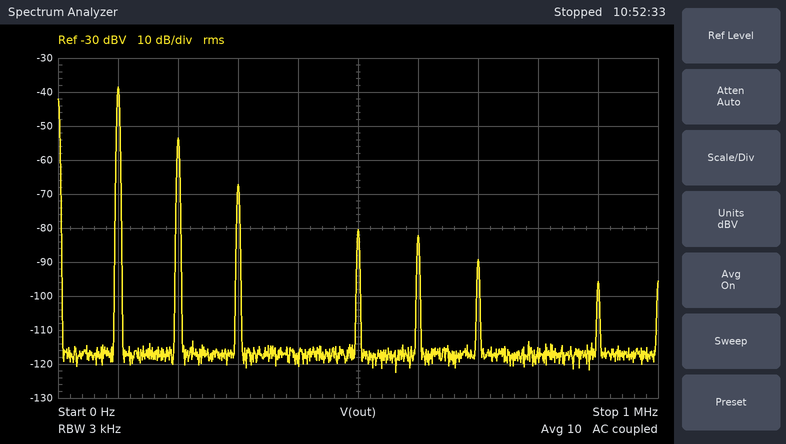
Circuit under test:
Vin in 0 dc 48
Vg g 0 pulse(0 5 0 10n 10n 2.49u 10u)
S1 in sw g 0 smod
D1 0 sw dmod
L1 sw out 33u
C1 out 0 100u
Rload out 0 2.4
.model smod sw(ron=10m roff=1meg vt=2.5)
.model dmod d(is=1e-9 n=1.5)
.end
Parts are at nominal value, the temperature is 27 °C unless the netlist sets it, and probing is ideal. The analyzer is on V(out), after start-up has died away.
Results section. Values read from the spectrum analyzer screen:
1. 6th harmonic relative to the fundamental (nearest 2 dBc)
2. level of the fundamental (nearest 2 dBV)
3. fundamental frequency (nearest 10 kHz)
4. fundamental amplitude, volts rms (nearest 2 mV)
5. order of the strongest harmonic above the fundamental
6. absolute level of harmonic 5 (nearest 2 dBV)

-44 dBc
-38 dBV
100 kHz
12 mV
2
-80 dBV
